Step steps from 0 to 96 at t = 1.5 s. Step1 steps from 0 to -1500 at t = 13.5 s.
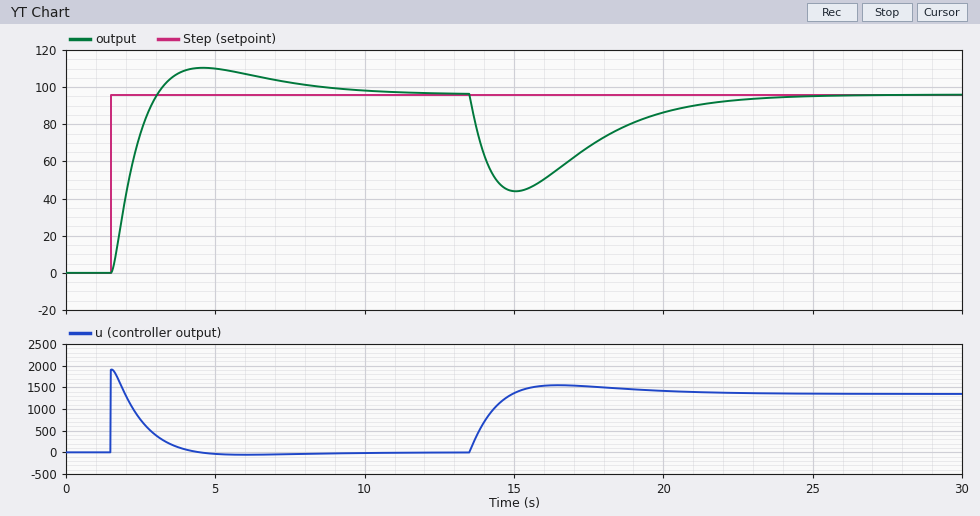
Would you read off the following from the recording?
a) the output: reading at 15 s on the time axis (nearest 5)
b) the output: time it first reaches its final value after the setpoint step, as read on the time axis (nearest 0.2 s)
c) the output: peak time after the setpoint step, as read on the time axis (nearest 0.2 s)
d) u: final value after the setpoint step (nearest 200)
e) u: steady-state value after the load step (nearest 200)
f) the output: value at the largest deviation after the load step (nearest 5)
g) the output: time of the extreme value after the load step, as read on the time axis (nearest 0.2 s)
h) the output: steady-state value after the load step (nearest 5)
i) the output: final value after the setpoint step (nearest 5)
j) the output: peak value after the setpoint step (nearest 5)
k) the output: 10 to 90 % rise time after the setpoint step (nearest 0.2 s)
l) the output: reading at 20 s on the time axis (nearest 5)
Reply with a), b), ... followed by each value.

a) 45
b) 3.0 s
c) 4.6 s
d) 0
e) 1400
f) 45
g) 15.0 s
h) 95
i) 95
j) 110
k) 1.0 s
l) 85
